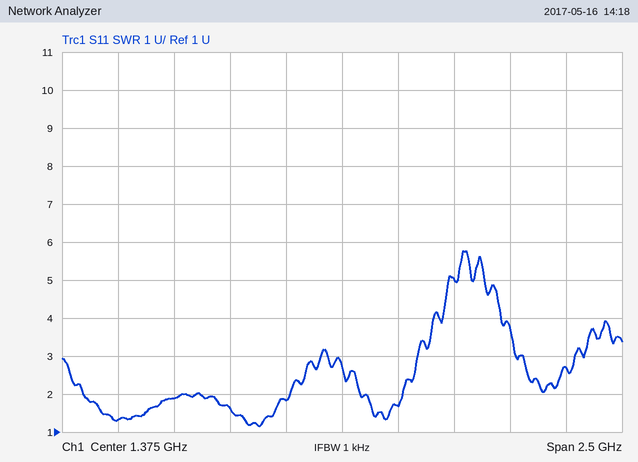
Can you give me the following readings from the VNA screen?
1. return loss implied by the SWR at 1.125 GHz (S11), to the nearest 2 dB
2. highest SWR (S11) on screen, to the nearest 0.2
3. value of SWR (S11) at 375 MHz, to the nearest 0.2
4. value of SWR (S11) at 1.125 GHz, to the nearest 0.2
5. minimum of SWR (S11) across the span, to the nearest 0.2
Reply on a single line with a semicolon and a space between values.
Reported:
10 dB; 5.8; 1.4; 1.8; 1.2
